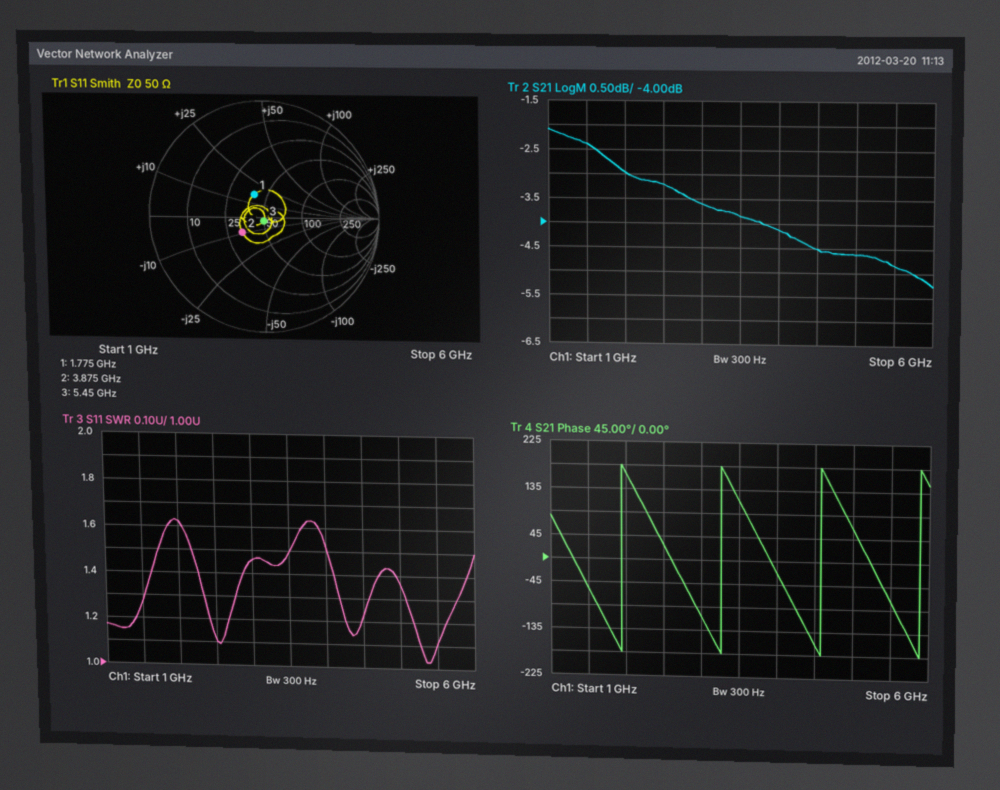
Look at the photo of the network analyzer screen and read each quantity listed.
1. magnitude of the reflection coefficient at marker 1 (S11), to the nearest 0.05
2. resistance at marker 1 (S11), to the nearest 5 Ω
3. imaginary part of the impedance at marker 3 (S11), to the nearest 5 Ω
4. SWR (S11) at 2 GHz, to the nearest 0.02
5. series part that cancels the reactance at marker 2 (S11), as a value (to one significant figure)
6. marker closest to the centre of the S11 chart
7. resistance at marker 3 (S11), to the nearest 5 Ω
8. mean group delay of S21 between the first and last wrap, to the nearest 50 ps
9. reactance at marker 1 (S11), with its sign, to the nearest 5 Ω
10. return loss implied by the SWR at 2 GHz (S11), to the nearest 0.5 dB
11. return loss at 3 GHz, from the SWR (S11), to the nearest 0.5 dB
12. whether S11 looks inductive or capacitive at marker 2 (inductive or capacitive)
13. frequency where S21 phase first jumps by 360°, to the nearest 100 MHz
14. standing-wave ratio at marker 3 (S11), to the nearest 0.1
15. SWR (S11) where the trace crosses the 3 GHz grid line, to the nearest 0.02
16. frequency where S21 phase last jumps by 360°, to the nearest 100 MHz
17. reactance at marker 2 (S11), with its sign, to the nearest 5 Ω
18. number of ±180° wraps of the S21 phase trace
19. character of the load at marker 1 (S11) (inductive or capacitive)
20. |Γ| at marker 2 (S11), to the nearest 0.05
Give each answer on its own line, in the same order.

0.20
40 Ω
-5 Ω
1.62
400 pH
marker 3
50 Ω
750 ps
+15 Ω
12.5 dB
14.5 dB
capacitive
1.9 GHz
1.1
1.46
5.9 GHz
-10 Ω
4
inductive
0.25
